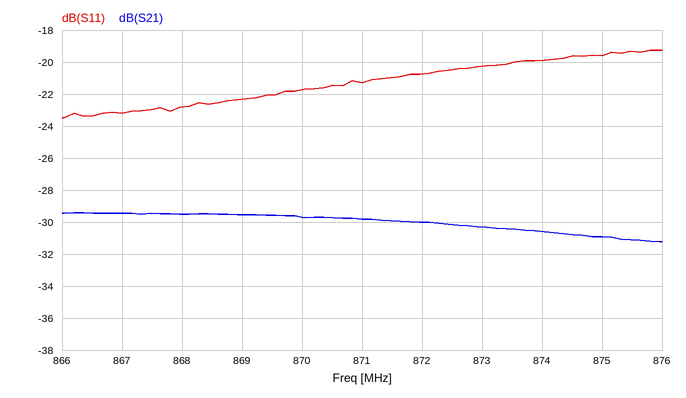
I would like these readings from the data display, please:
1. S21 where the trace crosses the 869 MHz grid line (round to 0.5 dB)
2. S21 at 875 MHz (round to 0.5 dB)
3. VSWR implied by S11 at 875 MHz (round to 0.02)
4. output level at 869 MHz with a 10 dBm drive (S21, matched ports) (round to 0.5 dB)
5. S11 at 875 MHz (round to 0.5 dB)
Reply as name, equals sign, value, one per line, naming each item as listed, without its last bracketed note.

S21 where the trace crosses the 869 MHz grid line = -29.5 dB
S21 at 875 MHz = -31.0 dB
VSWR implied by S11 at 875 MHz = 1.24
output level at 869 MHz with a 10 dBm drive (S21, matched ports) = -19.5 dBm
S11 at 875 MHz = -19.5 dB
